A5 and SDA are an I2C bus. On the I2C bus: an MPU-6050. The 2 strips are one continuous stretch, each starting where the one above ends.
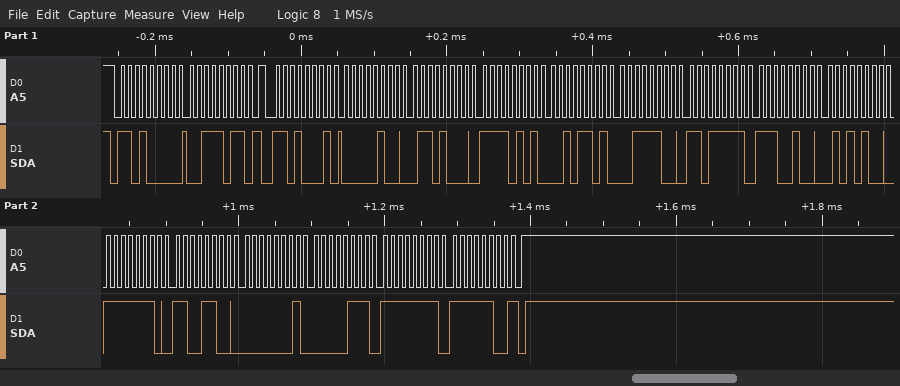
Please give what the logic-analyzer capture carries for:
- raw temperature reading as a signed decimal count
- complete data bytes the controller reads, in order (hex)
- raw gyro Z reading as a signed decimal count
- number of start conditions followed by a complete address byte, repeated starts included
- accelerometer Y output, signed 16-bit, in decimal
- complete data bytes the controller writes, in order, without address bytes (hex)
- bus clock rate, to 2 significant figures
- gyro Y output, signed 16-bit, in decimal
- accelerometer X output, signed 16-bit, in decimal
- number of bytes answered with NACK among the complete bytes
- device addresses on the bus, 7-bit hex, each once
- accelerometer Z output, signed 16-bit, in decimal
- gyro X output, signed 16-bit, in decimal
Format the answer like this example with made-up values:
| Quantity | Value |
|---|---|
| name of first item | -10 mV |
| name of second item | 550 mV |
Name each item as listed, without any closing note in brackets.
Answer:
| Quantity | Value |
|---|---|
| raw temperature reading as a signed decimal count | -7084 |
| complete data bytes the controller reads, in order | 04 68 F5 2D 3C DF E4 54 FE CC 01 07 FF FC |
| raw gyro Z reading as a signed decimal count | -4 |
| number of start conditions followed by a complete address byte, repeated starts included | 2 |
| accelerometer Y output, signed 16-bit, in decimal | -2771 |
| complete data bytes the controller writes, in order, without address bytes | 3B |
| bus clock rate, to 2 significant figures | 100 kHz |
| gyro Y output, signed 16-bit, in decimal | 263 |
| accelerometer X output, signed 16-bit, in decimal | 1128 |
| number of bytes answered with NACK among the complete bytes | 1 |
| device addresses on the bus, 7-bit hex, each once | 0x68 |
| accelerometer Z output, signed 16-bit, in decimal | 15583 |
| gyro X output, signed 16-bit, in decimal | -308 |
